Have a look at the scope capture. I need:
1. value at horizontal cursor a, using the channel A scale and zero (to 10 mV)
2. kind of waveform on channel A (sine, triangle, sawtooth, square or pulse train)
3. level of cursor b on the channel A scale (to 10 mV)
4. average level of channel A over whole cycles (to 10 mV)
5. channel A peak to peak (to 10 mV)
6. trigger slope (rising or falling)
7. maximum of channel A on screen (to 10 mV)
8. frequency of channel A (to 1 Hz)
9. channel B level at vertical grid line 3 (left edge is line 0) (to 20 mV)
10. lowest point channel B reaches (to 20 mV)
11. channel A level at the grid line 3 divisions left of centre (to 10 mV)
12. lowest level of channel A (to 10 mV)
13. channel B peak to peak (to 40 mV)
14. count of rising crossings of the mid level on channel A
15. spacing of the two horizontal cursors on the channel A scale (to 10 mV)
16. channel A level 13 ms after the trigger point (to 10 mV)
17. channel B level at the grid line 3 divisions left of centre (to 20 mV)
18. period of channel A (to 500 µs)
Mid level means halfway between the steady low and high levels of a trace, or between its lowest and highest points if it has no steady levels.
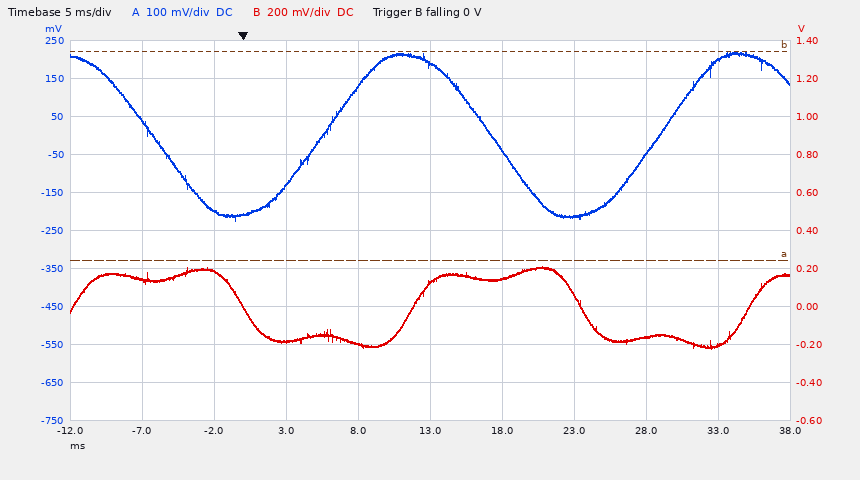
-330 mV
sine
220 mV
0 mV
440 mV
falling
220 mV
43 Hz
-180 mV
-220 mV
-200 mV
-220 mV
440 mV
2
550 mV
190 mV
180 mV
23.5 ms
